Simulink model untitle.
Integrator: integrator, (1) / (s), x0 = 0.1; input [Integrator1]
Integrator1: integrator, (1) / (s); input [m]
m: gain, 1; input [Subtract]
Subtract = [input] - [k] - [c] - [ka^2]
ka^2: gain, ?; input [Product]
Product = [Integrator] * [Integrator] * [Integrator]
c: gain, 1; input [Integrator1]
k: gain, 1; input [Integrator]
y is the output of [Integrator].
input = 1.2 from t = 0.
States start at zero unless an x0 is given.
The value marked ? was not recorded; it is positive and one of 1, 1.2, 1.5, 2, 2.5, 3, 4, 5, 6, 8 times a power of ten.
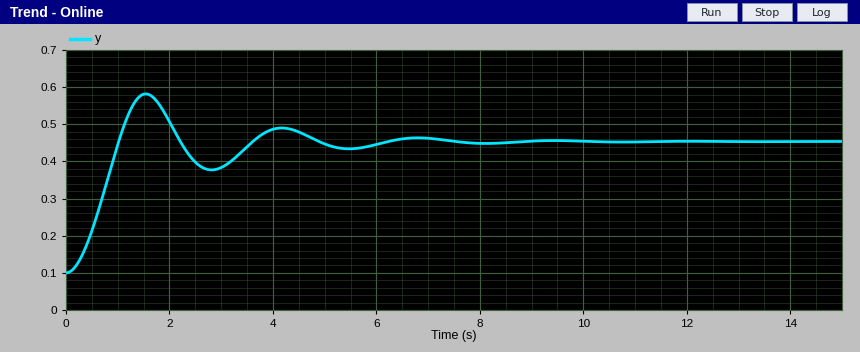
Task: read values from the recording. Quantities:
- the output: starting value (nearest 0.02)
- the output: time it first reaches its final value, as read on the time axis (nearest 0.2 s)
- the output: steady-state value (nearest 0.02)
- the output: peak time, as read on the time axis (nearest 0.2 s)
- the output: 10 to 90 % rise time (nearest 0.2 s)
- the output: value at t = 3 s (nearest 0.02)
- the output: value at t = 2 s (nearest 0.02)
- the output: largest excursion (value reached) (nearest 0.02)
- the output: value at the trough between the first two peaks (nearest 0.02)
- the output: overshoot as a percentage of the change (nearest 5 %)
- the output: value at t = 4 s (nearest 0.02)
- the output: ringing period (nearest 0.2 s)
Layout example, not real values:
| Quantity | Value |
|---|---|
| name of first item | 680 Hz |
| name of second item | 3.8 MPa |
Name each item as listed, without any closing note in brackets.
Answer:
| Quantity | Value |
|---|---|
| the output: starting value | 0.10 |
| the output: time it first reaches its final value, as read on the time axis | 1.0 s |
| the output: steady-state value | 0.46 |
| the output: peak time, as read on the time axis | 1.6 s |
| the output: 10 to 90 % rise time | 0.6 s |
| the output: value at t = 3 s | 0.38 |
| the output: value at t = 2 s | 0.50 |
| the output: largest excursion (value reached) | 0.58 |
| the output: value at the trough between the first two peaks | 0.38 |
| the output: overshoot as a percentage of the change | 35 % |
| the output: value at t = 4 s | 0.48 |
| the output: ringing period | 2.6 s |
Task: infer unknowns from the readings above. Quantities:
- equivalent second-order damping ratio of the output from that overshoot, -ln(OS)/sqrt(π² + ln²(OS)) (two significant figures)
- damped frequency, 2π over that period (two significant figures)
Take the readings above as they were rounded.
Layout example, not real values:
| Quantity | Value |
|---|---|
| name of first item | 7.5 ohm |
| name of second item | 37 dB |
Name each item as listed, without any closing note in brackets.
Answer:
| Quantity | Value |
|---|---|
| equivalent second-order damping ratio of the output from that overshoot, -ln(OS)/sqrt(π² + ln²(OS)) | 0.32 |
| damped frequency, 2π over that period | 2.4 rad/s |
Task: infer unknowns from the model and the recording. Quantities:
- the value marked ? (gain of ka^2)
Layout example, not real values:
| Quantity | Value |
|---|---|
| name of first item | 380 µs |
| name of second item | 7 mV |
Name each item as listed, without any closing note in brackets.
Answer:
| Quantity | Value |
|---|---|
| the value marked ? | 8 |
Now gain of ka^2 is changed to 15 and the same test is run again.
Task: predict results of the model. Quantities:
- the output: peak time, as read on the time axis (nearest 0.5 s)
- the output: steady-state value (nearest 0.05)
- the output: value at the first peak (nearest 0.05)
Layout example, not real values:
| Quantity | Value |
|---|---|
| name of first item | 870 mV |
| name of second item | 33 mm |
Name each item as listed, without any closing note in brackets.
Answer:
| Quantity | Value |
|---|---|
| the output: peak time, as read on the time axis | 1.5 s |
| the output: steady-state value | 0.40 |
| the output: value at the first peak | 0.50 |
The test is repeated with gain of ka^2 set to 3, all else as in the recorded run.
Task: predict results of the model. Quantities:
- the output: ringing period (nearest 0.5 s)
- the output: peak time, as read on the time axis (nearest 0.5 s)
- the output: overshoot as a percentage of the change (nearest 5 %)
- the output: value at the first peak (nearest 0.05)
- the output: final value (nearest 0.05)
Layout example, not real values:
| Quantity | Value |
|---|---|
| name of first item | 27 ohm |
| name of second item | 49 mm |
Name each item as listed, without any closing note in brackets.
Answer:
| Quantity | Value |
|---|---|
| the output: ringing period | 3.0 s |
| the output: peak time, as read on the time axis | 2.0 s |
| the output: overshoot as a percentage of the change | 30 % |
| the output: value at the first peak | 0.75 |
| the output: final value | 0.60 |
